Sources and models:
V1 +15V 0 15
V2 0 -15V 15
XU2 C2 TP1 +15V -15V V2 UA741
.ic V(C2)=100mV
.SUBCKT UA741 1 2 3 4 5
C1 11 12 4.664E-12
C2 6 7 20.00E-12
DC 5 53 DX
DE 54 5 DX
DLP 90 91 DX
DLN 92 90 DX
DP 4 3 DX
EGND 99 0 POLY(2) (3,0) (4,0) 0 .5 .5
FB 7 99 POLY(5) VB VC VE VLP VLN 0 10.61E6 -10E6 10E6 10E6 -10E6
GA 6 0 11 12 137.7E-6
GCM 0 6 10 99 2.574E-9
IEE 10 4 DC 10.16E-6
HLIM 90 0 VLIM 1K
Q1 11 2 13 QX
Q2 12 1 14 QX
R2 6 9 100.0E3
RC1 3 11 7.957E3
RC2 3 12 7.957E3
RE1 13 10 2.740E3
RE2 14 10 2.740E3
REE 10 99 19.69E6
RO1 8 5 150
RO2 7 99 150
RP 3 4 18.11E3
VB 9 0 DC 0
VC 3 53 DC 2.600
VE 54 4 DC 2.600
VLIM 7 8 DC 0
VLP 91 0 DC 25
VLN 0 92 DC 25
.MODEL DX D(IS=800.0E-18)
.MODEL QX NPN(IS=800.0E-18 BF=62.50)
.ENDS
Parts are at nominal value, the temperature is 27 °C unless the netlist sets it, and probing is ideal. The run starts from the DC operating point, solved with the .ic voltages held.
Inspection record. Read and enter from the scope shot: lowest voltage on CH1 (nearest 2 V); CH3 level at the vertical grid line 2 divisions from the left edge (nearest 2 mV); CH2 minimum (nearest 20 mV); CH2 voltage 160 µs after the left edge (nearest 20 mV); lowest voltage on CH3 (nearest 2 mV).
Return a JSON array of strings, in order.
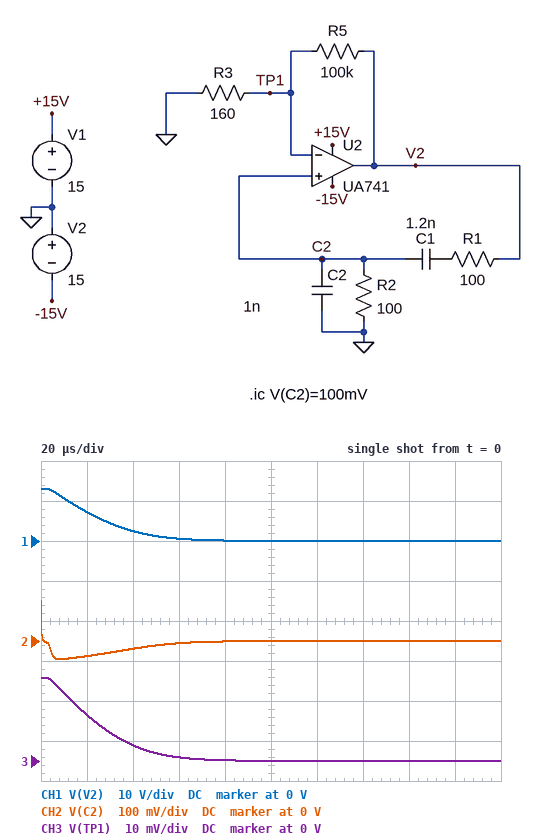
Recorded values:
["0 V", "4 mV", "-40 mV", "0 V", "0 V"]
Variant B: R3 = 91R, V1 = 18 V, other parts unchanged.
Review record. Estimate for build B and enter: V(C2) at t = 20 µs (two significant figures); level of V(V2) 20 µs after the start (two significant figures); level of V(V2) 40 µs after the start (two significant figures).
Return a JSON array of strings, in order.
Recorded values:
["-34 mV", "11 V", "6.4 V"]
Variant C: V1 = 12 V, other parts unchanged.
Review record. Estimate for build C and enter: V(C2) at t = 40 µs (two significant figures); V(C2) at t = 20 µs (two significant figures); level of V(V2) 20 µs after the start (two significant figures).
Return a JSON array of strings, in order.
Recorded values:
["-13 mV", "-32 mV", "5.1 V"]
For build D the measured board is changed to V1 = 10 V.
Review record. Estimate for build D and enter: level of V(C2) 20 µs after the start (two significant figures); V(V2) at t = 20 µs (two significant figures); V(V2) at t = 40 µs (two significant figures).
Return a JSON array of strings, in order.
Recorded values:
["-27 mV", "3.8 V", "910 mV"]
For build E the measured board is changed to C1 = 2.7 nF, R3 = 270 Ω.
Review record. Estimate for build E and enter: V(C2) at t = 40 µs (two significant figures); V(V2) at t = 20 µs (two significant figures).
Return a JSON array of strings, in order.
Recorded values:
["-140 mV", "3.9 V"]
